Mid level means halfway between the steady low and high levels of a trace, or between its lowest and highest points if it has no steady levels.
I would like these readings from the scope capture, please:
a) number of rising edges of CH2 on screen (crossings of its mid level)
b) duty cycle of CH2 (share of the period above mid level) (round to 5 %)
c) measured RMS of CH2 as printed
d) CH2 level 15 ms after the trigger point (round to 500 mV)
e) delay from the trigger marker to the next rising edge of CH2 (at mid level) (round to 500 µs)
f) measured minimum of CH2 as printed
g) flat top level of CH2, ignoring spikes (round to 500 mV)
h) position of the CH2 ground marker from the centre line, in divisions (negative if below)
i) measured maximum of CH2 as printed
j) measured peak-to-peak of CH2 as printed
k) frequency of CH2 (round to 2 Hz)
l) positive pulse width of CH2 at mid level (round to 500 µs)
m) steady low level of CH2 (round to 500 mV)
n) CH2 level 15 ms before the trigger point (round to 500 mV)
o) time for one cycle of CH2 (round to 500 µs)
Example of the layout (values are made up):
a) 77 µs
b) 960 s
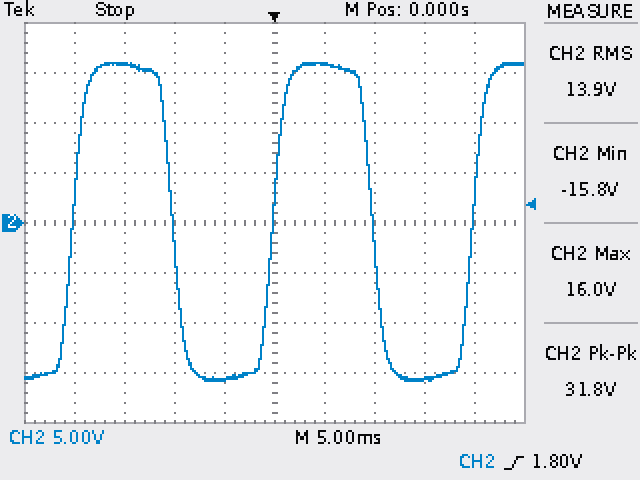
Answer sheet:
a) 3
b) 50 %
c) 13.9 V
d) -15.5 V
e) 20.0 ms
f) -15.8 V
g) 16.0 V
h) 0.0 div
i) 16.0 V
j) 31.8 V
k) 50 Hz
l) 10.0 ms
m) -15.5 V
n) 16.0 V
o) 20.0 ms
